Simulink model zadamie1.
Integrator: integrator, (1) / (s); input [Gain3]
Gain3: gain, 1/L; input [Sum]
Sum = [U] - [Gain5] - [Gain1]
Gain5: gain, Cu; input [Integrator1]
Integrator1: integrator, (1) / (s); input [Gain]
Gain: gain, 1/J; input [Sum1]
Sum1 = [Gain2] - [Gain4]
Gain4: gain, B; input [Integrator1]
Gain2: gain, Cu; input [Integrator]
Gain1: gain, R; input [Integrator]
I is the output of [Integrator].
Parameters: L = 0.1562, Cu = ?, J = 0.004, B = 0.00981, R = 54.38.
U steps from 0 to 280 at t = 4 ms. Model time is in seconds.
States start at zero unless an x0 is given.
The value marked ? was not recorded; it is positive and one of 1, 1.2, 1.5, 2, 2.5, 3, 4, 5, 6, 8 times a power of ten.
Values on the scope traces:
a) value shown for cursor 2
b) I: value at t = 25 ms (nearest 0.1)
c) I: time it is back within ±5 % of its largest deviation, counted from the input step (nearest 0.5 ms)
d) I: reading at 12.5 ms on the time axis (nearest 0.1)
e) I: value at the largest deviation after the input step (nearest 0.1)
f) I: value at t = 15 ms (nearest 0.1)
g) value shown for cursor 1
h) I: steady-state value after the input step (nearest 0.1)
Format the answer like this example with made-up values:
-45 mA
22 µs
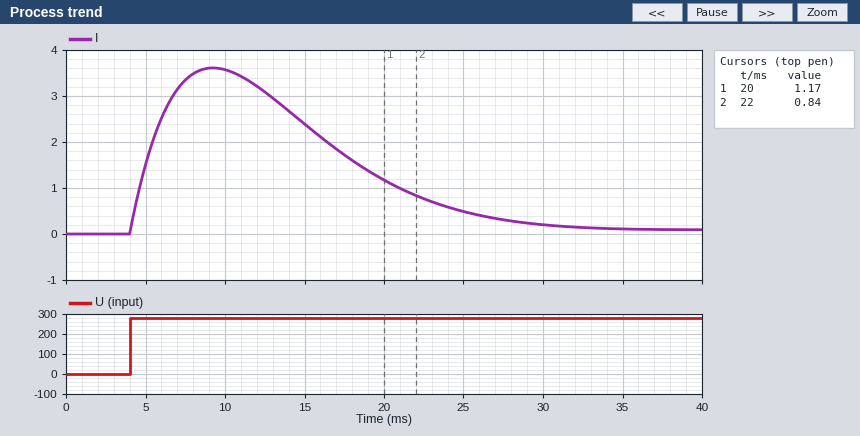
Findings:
0.84
0.5
24.0 ms
3.1
3.6
2.4
1.17
0.1
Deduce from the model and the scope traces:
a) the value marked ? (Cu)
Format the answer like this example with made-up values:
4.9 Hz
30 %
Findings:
5
